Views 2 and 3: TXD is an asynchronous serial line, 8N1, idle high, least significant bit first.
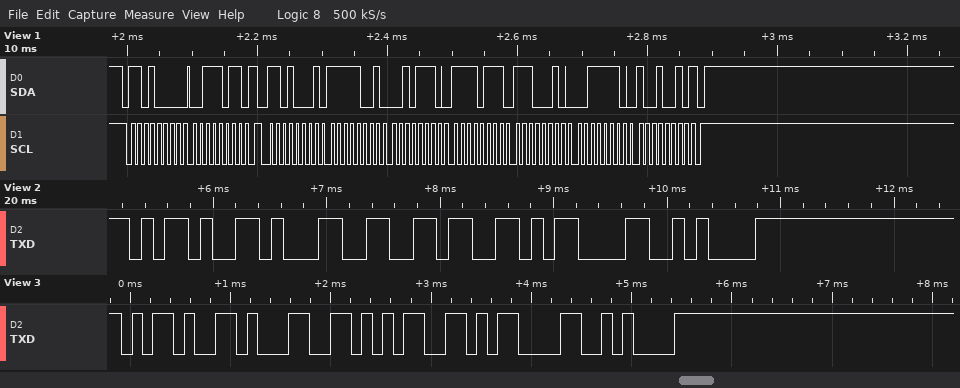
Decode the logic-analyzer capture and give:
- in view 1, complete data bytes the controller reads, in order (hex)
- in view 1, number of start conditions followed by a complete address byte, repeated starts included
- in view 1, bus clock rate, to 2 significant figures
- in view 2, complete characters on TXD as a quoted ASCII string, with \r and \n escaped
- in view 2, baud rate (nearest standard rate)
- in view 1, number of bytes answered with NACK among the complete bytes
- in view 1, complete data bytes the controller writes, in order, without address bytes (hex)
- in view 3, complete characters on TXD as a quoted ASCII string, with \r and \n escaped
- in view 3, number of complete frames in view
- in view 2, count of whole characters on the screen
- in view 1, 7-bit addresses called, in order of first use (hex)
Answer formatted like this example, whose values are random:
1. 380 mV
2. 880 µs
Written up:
1. F9 2E F7 E2 3E 92
2. 2
3. 100 kHz
4. "-16\r\n"
5. 9600 baud
6. 1
7. 3B
8. "-15\r\n"
9. 5
10. 5
11. 0x68
